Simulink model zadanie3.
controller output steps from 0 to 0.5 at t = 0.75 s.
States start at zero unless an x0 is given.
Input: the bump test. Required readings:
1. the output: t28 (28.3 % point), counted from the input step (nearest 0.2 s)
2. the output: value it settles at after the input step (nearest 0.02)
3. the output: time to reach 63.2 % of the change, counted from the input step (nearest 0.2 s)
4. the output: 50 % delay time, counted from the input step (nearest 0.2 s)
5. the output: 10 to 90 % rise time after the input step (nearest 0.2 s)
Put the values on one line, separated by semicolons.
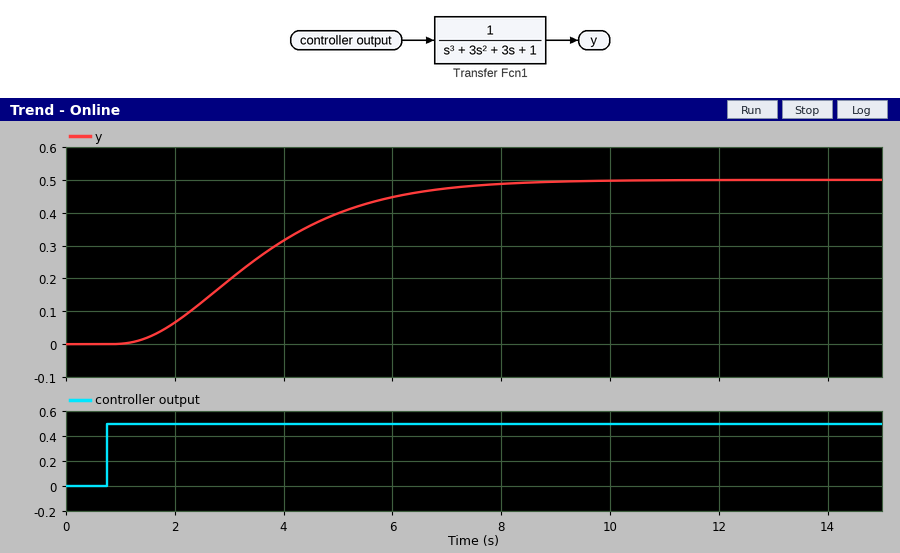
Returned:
1.8 s; 0.50; 3.2 s; 2.6 s; 4.2 s
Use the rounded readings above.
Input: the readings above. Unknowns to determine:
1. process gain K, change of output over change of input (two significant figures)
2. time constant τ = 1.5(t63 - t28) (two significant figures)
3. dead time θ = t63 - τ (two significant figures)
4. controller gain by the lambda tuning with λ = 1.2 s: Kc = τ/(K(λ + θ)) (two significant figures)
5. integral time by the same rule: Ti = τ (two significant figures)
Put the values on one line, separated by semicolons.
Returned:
1.0; 2.1 s; 1.1 s; 0.91; 2.1 s
